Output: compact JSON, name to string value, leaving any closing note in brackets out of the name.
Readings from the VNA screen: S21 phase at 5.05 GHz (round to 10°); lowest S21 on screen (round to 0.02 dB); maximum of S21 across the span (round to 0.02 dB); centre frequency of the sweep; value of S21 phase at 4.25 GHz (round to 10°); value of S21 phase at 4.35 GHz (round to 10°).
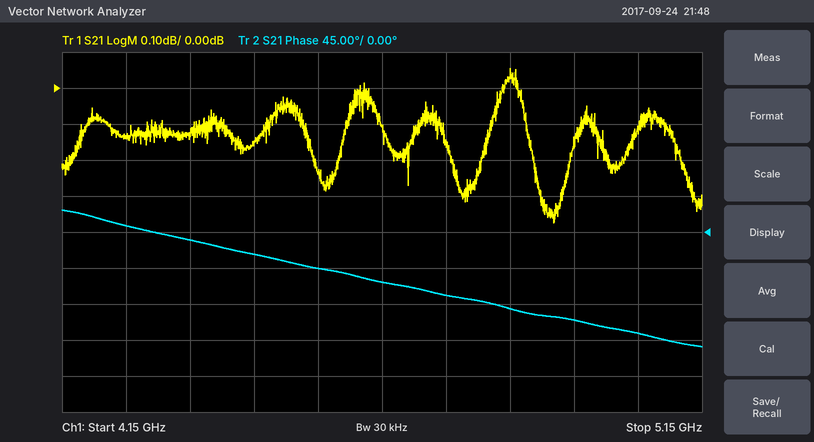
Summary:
{"S21 phase at 5.05 GHz": "-130°", "lowest S21 on screen": "-0.38 dB", "maximum of S21 across the span": "0.06 dB", "centre frequency of the sweep": "4.65 GHz", "value of S21 phase at 4.25 GHz": "10°", "value of S21 phase at 4.35 GHz": "-10°"}
